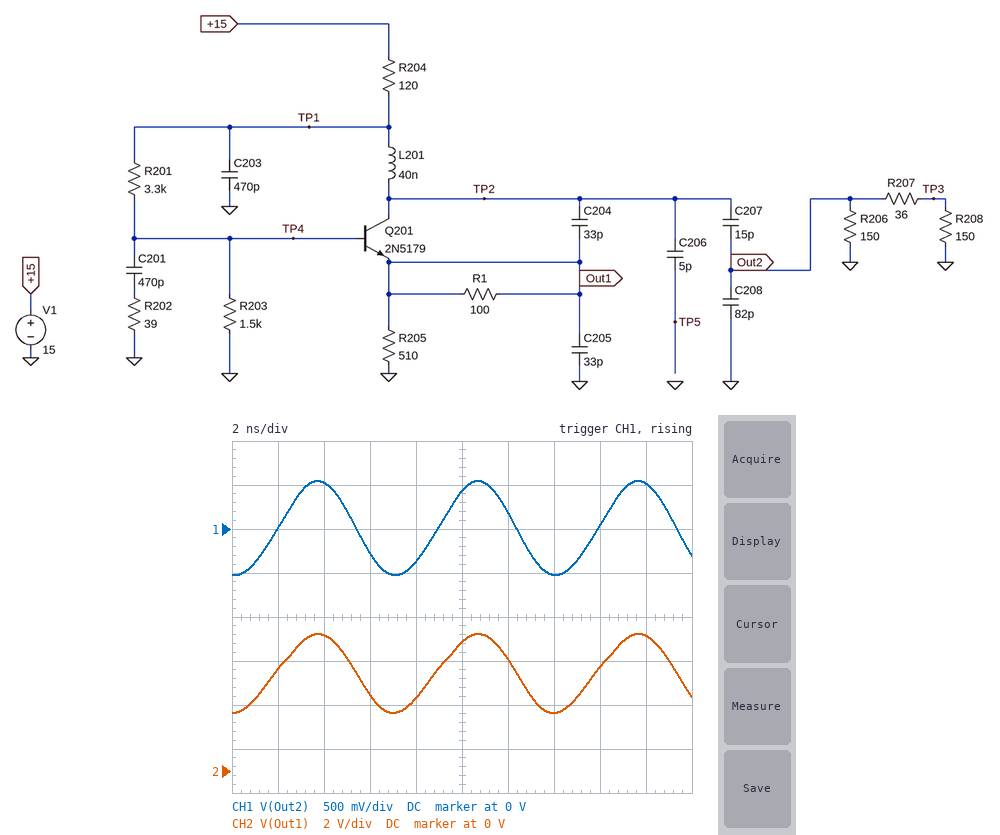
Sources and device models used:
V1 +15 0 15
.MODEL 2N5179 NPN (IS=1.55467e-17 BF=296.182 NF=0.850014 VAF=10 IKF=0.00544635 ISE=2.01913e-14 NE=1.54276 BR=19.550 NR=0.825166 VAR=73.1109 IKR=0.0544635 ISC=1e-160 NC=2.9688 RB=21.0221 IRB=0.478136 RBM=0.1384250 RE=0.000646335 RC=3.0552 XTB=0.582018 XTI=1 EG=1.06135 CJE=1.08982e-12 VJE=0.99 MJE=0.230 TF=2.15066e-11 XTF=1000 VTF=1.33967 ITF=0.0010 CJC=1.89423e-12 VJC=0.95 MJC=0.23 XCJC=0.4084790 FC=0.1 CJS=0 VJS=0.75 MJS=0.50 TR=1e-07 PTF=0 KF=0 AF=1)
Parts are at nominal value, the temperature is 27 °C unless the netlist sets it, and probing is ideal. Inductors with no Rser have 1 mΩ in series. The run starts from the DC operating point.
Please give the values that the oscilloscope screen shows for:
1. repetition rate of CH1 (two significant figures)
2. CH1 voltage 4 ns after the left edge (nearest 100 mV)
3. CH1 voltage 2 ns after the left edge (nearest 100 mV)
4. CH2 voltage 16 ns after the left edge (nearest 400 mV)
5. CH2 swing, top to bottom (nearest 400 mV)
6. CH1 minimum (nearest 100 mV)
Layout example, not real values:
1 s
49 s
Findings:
140 MHz
500 mV
0 V
4.8 V
3.6 V
-500 mV
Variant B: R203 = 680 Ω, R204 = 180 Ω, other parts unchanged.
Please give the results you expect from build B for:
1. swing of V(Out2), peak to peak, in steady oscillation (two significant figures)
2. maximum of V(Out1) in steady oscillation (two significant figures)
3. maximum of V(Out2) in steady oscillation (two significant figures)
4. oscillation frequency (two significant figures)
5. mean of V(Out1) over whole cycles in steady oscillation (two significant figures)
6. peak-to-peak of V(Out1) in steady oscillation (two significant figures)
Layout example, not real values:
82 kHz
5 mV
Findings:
1.2 V
5.0 V
630 mV
150 MHz
3.0 V
4.1 V
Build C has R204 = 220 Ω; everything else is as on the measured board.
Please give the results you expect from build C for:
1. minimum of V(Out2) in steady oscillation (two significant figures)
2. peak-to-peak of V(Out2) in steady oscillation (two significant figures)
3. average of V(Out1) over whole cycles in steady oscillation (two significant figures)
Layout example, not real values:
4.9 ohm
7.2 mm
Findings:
-430 mV
880 mV
4.0 V
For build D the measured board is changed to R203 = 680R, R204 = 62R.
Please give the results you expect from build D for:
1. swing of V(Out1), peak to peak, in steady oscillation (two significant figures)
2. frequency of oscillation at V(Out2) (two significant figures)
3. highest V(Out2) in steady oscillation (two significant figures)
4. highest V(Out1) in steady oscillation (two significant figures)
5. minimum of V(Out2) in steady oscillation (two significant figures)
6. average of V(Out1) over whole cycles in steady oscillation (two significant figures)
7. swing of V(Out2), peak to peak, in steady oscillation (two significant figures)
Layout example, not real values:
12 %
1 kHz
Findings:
4.7 V
150 MHz
720 mV
5.7 V
-690 mV
3.4 V
1.4 V
